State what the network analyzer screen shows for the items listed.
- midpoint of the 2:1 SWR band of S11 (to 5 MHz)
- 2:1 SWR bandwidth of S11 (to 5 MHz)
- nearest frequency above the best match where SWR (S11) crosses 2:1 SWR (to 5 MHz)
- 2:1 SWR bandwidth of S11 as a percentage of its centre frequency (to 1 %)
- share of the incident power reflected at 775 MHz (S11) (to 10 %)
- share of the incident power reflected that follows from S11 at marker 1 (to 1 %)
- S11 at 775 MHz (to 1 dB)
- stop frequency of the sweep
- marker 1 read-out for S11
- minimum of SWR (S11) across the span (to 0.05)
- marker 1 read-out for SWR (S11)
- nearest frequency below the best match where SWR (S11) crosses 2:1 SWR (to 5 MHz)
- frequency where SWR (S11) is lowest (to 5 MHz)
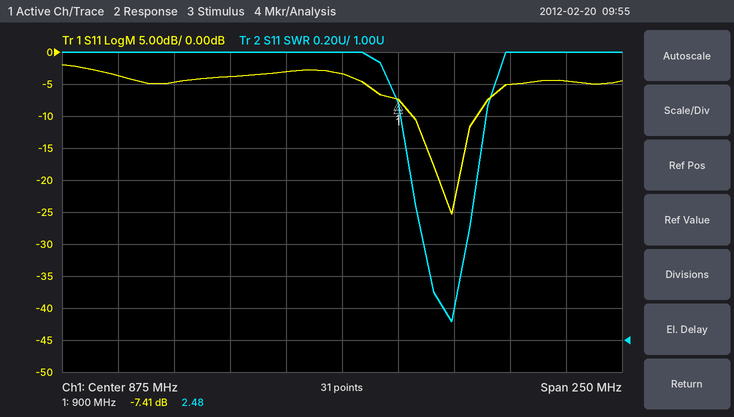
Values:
920 MHz
30 MHz
935 MHz
3 %
40 %
18 %
-4 dB
1 GHz
-7.41 dB
1.10
2.48
905 MHz
925 MHz
